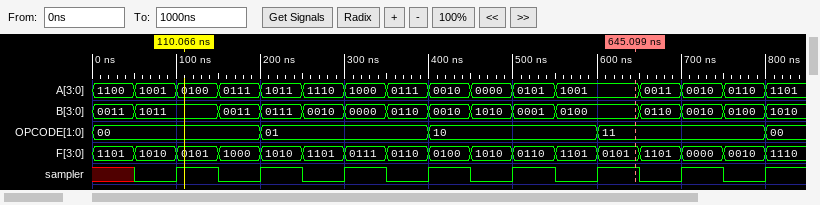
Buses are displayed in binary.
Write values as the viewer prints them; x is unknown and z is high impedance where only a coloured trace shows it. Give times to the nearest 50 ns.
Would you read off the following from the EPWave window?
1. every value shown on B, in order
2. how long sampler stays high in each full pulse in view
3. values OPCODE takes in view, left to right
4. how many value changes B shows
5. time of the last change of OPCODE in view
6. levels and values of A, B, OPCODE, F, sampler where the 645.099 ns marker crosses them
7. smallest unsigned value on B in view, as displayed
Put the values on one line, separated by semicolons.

0011, 1011, 0011, 0111, 0010, 0000, 0110, 0010, 1010, 0001, 0100, 0110, 0010, 0100, 1010; 50 ns, 50 ns, 50 ns, 50 ns, 50 ns, 50 ns, 50 ns; 00, 01, 10, 11, 00; 14; 800 ns; A=1001, B=0100, OPCODE=11, F=0101, sampler=1; 0000
